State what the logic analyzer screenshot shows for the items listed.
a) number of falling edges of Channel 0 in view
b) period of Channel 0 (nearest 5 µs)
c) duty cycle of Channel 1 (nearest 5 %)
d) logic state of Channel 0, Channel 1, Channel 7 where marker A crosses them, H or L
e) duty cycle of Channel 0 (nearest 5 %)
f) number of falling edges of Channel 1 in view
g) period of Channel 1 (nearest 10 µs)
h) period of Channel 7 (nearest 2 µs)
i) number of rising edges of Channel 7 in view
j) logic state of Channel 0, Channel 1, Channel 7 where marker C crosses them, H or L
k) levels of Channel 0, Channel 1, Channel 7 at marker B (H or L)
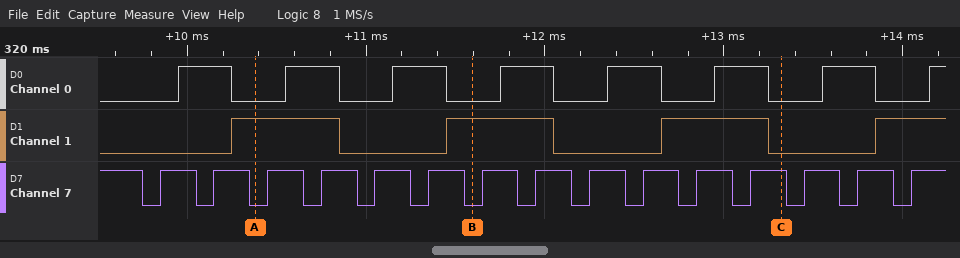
7
600 µs
50 %
Channel 0=L, Channel 1=H, Channel 7=L
50 %
3
1200 µs
300 µs
15
Channel 0=L, Channel 1=L, Channel 7=H
Channel 0=L, Channel 1=H, Channel 7=L
